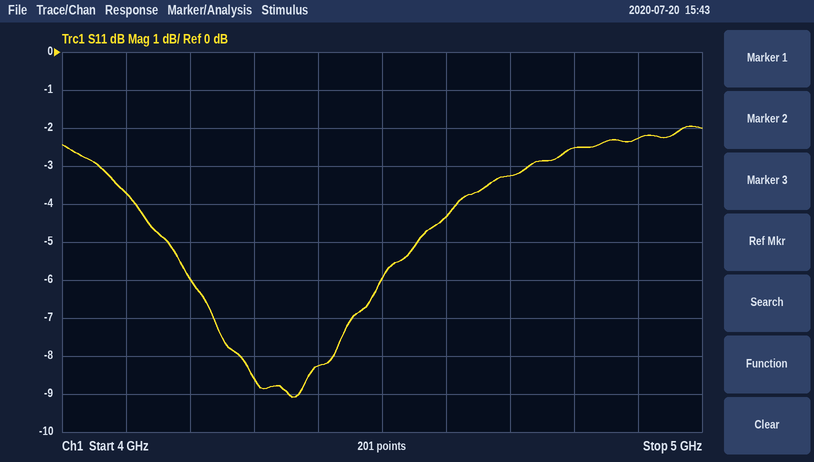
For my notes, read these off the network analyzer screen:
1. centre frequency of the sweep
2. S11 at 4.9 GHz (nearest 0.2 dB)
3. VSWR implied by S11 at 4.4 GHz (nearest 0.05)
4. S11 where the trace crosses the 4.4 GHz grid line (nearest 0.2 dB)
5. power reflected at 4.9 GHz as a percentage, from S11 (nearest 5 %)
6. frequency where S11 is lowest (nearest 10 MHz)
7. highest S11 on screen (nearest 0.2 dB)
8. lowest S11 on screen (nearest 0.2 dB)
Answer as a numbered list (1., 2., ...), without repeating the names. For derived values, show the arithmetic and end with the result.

1. 4.5 GHz
2. -2.2 dB
3. |Γ| = 10^(-8.2/20) = 0.3890; VSWR = (1 + 0.3890)/(1 − 0.3890) ≈ 2.27, so 2.25 to the nearest 0.05
4. -8.2 dB
5. 10^(-2.2/10) ≈ 60 %
6. 4.36 GHz
7. -2.0 dB
8. -9.0 dB
